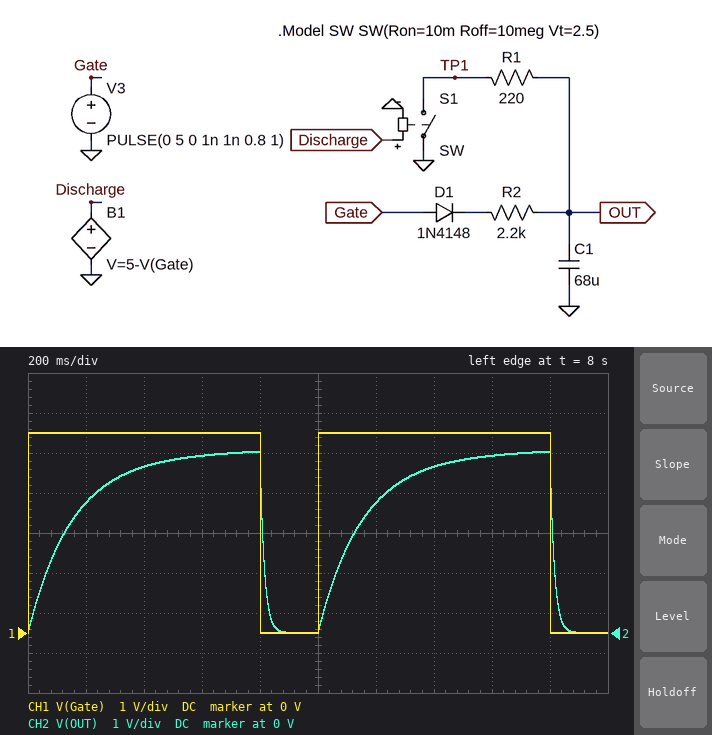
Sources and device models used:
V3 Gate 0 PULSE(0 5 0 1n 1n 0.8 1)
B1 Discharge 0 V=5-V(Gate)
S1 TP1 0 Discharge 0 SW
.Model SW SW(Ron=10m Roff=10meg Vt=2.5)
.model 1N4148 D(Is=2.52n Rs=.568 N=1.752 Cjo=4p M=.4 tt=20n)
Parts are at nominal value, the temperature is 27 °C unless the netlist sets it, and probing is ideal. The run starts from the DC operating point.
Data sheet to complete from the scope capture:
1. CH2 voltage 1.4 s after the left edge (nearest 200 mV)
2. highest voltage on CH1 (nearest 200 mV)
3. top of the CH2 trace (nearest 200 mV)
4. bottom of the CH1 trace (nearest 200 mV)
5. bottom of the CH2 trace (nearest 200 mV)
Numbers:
4.2 V
5.0 V
4.6 V
0 V
0 V
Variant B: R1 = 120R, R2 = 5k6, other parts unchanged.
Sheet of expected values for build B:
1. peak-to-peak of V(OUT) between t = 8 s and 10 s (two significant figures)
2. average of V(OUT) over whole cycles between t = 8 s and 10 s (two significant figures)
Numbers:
3.9 V
2.1 V
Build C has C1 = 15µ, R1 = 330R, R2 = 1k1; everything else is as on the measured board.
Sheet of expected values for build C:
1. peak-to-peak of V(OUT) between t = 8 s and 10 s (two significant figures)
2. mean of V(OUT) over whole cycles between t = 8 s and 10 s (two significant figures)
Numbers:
4.7 V
3.7 V
